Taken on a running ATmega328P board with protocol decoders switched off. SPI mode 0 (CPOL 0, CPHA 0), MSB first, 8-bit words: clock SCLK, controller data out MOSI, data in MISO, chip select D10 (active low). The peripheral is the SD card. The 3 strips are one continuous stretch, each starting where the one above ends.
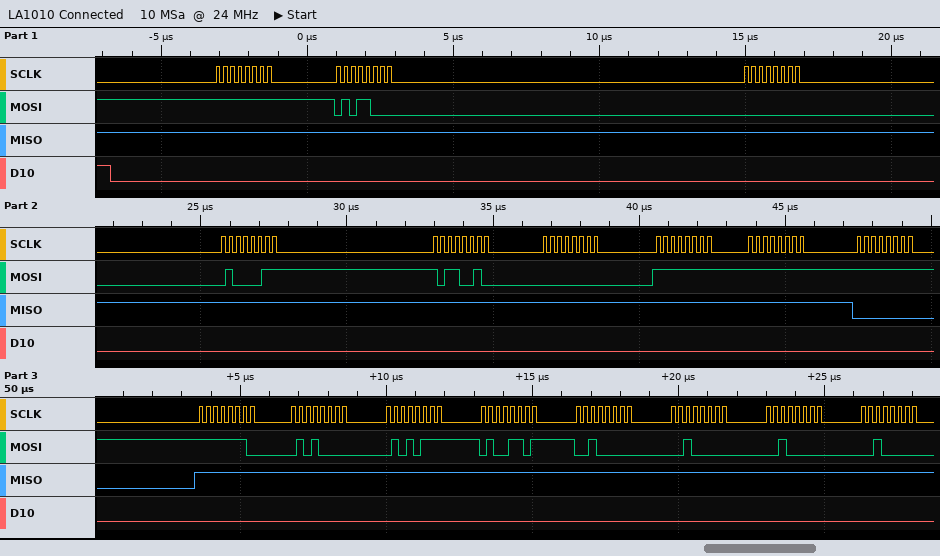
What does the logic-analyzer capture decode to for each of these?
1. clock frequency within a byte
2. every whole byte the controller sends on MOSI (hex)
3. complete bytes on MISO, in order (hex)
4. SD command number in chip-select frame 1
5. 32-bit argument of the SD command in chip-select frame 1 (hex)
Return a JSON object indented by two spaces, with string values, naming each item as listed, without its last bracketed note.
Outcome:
{
  "clock frequency within a byte": "4 MHz",
  "every whole byte the controller sends on MOSI": "FF 58 00 43 B2 00 FF FF FF FE 50 57 4D 20 20 20 20",
  "complete bytes on MISO, in order": "FF FF FF FF FF FF FF FF 00 FF FF FF FF FF FF FF FF",
  "SD command number in chip-select frame 1": "CMD24",
  "32-bit argument of the SD command in chip-select frame 1": "0x0043B200"
}
